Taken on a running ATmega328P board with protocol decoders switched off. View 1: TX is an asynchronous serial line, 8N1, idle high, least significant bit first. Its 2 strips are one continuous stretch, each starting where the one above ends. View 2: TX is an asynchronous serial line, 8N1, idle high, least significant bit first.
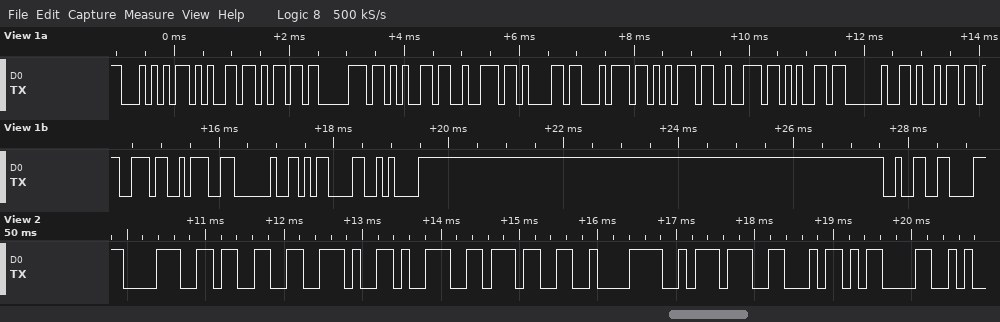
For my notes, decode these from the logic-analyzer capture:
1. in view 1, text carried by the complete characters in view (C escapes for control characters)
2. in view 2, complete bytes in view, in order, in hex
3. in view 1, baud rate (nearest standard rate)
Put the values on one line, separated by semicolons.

"Temperature is: \r\n2"; 0x38 0x33 0x2E 0x39 0x37 0xC2 0xBA 0x46 0x0D; 9600 baud
